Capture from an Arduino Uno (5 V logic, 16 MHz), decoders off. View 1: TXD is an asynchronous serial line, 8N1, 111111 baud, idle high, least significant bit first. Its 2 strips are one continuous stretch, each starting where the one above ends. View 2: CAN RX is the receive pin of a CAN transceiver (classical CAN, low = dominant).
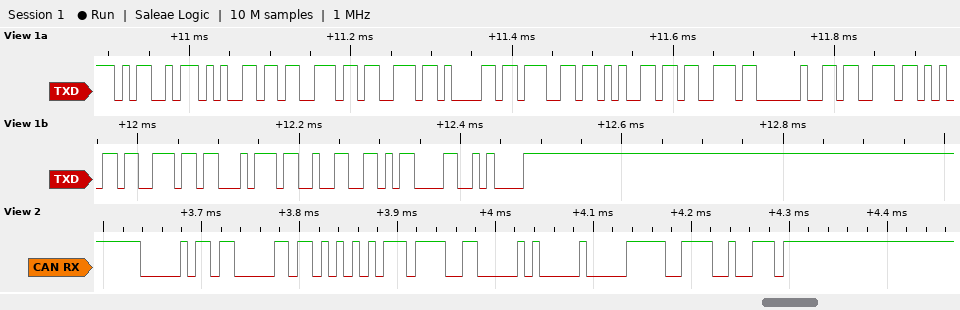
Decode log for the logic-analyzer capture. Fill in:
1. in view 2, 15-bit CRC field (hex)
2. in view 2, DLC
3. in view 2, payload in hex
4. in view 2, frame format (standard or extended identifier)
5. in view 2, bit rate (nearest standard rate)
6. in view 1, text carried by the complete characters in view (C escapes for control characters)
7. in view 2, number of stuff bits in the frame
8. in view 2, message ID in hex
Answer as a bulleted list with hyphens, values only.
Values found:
- 0x7793
- 5
- AA BB CC 08 01
- standard
- 125 kbit/s
- "Messages sent2\r\n"
- 6
- 0x036
